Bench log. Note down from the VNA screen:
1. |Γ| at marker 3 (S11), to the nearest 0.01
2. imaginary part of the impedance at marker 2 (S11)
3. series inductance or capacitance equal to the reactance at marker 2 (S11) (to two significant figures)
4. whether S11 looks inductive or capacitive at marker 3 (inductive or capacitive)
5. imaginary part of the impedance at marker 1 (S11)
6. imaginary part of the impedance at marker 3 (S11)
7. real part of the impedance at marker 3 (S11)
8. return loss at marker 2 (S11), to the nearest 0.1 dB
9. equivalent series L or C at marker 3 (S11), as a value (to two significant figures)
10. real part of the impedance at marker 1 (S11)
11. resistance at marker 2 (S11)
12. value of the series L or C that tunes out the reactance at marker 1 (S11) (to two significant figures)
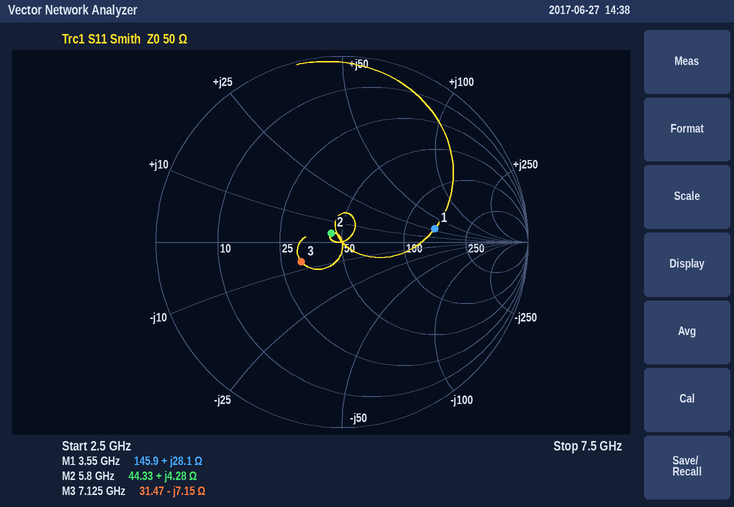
0.24
+4.28 Ω
120 pH
capacitive
+28.1 Ω
-7.15 Ω
31.47 Ω
22.5 dB
3.1 pF
145.9 Ω
44.33 Ω
1.6 pF
